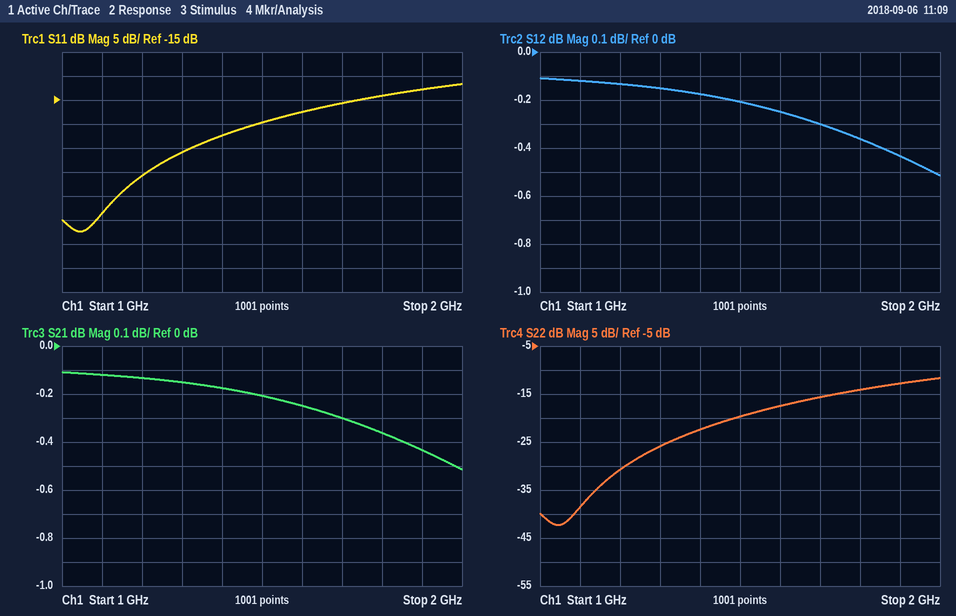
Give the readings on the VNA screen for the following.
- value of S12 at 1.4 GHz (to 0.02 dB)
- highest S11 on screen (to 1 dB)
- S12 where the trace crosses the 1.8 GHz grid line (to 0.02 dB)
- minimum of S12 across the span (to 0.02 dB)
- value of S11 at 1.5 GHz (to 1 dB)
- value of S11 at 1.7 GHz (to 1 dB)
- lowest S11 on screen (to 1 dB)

-0.18 dB
-12 dB
-0.36 dB
-0.52 dB
-20 dB
-16 dB
-42 dB
